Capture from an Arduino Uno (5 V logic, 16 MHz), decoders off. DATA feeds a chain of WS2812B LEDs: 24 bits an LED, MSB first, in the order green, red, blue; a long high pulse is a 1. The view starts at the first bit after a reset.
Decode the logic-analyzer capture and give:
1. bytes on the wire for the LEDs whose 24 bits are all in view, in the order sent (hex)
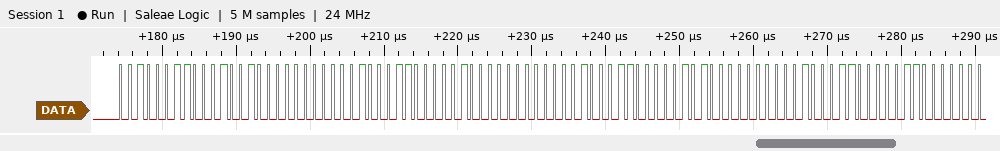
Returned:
23 12 00 23 04 00 23 05 00
